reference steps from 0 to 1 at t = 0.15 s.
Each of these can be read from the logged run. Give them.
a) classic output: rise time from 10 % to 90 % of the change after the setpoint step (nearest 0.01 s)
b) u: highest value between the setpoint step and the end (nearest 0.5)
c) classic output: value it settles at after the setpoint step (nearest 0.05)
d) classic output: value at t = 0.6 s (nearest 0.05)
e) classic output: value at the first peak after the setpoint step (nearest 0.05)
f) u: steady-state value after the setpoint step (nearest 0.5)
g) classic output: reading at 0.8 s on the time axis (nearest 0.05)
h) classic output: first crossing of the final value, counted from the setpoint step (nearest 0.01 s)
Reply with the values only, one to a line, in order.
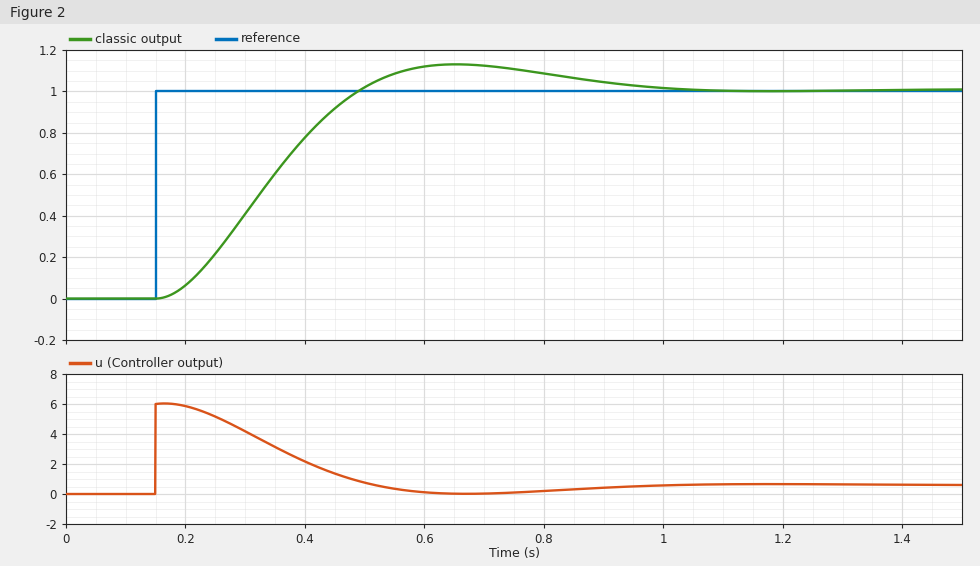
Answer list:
0.23 s
6.0
1.00
1.10
1.15
0.5
1.10
0.34 s
